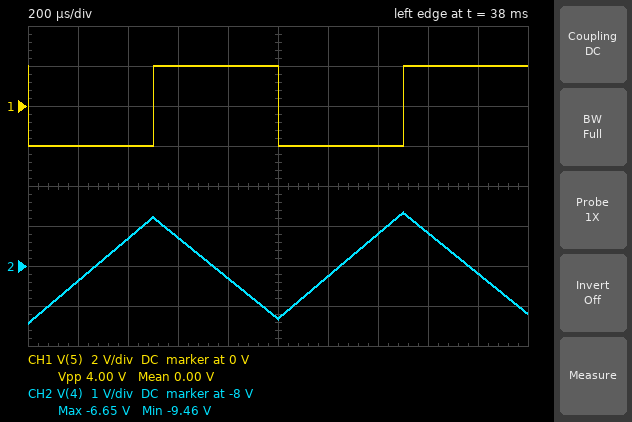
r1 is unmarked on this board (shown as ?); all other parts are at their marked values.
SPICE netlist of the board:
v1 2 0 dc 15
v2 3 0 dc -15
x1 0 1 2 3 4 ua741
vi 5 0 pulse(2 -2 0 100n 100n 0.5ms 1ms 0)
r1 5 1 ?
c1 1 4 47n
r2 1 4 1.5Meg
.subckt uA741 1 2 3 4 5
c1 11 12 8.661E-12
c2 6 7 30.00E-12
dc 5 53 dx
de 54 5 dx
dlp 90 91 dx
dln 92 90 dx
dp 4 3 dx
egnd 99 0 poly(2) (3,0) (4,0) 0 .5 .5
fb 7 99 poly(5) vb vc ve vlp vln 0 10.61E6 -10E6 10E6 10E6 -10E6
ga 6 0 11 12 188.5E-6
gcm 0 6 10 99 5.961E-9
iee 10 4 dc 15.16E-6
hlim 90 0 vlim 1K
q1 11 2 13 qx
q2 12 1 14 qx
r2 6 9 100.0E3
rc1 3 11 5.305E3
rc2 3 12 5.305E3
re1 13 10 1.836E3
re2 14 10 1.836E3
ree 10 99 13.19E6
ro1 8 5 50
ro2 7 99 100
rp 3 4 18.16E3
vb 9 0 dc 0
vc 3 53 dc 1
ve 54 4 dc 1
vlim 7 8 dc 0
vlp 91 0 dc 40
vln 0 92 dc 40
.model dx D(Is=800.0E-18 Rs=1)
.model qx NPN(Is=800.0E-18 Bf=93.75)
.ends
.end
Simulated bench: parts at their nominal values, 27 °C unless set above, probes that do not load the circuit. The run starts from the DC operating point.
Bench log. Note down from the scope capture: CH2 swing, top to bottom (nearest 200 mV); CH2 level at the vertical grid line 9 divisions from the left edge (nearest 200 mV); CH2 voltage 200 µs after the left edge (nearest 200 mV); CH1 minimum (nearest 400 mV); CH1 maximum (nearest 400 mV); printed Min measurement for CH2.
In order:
2.8 V
-8.2 V
-8.4 V
-2.0 V
2.0 V
-9.46 V
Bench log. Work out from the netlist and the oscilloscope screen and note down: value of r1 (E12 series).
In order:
8.2 kΩ
